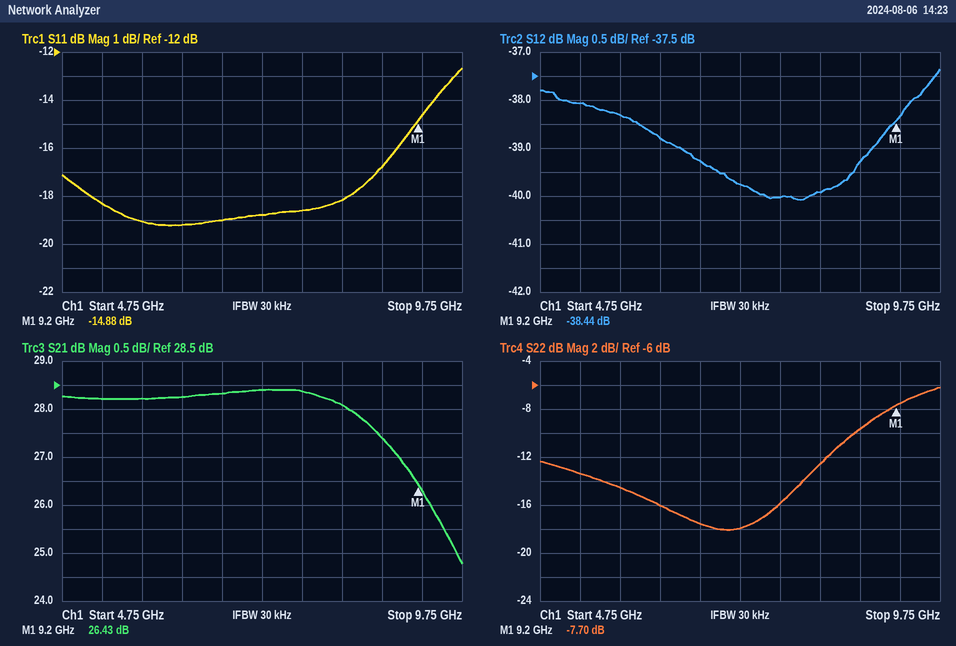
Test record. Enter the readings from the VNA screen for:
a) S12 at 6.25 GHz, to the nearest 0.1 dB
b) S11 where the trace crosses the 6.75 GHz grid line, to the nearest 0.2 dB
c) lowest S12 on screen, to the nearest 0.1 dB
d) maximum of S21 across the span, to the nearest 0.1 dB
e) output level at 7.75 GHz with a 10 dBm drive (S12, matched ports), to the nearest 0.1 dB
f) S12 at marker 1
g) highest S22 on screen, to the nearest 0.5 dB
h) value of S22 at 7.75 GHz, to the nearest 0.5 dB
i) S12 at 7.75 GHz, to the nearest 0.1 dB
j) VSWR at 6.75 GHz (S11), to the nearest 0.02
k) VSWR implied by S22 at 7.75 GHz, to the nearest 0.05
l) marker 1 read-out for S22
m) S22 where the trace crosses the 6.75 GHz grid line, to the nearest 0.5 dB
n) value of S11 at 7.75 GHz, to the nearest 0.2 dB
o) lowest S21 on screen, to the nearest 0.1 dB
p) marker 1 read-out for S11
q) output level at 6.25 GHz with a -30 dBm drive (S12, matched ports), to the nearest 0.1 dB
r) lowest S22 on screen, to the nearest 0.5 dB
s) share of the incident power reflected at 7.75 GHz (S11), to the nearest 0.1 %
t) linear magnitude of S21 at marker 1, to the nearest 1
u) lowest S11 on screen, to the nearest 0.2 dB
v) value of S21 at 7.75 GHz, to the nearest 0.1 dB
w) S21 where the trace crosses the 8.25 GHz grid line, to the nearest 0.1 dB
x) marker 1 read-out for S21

-38.8 dB
-19.0 dB
-40.1 dB
28.4 dB
-30.0 dBm
-38.44 dB
-6.0 dB
-16.0 dB
-40.0 dB
1.26
1.40
-7.70 dB
-17.5 dB
-18.6 dB
24.8 dB
-14.88 dB
-68.8 dBm
-18.0 dB
1.4 %
21
-19.2 dB
28.4 dB
28.1 dB
26.43 dB
